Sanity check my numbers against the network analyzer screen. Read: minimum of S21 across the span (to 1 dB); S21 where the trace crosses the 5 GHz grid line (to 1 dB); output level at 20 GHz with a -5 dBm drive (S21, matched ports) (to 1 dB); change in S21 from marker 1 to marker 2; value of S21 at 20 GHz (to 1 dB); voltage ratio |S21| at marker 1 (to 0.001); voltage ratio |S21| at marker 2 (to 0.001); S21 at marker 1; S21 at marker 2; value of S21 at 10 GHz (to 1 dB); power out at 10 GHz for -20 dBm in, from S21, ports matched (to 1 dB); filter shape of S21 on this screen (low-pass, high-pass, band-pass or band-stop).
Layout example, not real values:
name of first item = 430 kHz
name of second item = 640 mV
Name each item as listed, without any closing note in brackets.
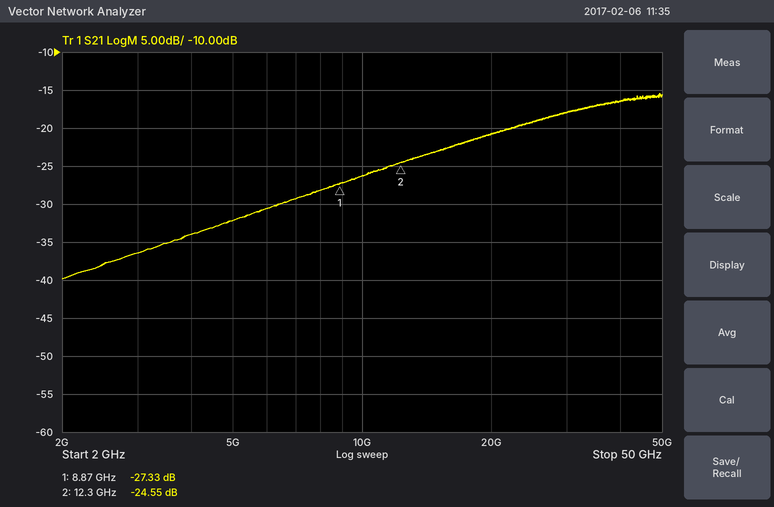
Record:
minimum of S21 across the span = -40 dB
S21 where the trace crosses the 5 GHz grid line = -32 dB
output level at 20 GHz with a -5 dBm drive (S21, matched ports) = -26 dBm
change in S21 from marker 1 to marker 2 = 2.78 dB
value of S21 at 20 GHz = -21 dB
voltage ratio |S21| at marker 1 = 0.043
voltage ratio |S21| at marker 2 = 0.059
S21 at marker 1 = -27.33 dB
S21 at marker 2 = -24.55 dB
value of S21 at 10 GHz = -26 dB
power out at 10 GHz for -20 dBm in, from S21, ports matched = -46 dBm
filter shape of S21 on this screen = high-pass
